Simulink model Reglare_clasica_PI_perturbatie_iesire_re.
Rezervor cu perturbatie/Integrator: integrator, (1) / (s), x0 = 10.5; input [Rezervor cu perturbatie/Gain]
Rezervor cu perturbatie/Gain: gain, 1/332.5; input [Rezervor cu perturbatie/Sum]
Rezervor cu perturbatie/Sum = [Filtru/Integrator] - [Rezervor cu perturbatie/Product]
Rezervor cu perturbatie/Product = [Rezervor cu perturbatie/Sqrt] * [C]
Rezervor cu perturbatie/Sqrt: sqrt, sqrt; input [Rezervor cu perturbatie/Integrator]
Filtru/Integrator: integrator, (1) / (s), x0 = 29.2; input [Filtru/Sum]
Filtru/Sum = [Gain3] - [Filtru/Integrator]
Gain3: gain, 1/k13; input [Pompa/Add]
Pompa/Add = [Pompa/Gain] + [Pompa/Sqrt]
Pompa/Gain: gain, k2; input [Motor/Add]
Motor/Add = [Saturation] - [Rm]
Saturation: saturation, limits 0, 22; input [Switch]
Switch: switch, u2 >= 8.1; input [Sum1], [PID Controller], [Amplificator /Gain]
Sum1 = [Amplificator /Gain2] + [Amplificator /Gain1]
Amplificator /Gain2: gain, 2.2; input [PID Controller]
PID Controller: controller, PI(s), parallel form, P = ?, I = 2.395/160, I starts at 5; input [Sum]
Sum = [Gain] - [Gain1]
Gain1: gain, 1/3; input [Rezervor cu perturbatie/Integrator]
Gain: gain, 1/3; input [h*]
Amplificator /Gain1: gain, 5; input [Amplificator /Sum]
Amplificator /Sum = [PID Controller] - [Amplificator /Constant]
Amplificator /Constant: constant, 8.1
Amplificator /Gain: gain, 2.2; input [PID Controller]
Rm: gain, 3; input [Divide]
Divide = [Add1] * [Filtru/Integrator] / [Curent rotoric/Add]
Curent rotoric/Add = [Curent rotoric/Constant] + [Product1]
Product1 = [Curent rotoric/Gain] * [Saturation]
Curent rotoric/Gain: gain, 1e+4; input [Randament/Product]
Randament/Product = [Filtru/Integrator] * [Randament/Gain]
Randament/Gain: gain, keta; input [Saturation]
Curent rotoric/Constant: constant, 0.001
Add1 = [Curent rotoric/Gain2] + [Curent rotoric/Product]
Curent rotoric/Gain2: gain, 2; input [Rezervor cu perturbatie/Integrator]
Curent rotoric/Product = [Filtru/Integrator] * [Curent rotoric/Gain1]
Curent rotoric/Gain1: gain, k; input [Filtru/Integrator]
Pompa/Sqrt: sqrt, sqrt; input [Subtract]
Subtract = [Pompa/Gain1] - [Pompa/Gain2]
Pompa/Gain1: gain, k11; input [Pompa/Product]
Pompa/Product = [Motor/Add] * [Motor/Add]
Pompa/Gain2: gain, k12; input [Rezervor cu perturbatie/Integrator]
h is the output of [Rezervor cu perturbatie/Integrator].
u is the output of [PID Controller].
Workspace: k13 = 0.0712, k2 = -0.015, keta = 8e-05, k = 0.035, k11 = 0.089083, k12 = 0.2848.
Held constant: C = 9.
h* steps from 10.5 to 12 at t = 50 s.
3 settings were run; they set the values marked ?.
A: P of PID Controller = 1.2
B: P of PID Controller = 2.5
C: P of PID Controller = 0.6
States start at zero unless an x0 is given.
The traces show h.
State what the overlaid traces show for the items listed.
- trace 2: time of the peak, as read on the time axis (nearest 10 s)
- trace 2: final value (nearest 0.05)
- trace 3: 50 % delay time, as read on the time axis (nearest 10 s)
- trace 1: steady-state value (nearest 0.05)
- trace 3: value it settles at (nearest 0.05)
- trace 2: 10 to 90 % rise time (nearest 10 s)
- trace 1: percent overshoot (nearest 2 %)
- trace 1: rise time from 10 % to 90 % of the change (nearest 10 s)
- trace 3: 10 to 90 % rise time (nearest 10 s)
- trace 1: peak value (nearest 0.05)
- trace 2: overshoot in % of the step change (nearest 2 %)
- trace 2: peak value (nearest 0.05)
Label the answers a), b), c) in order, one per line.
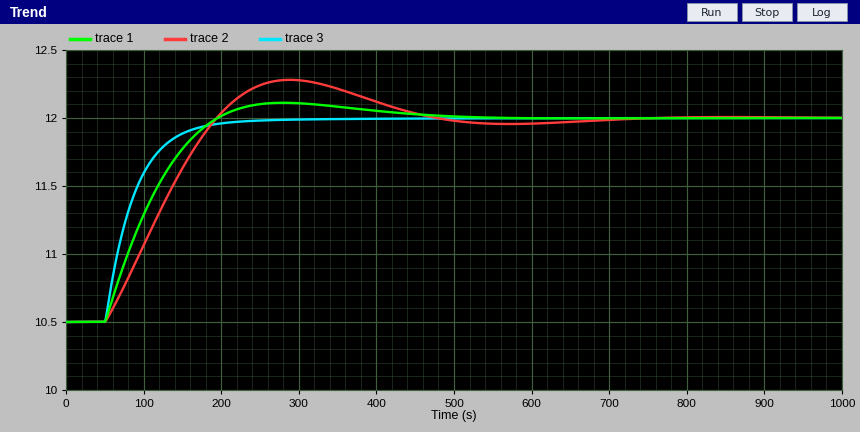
a) 290 s
b) 12.00
c) 80 s
d) 12.00
e) 12.00
f) 110 s
g) 8 %
h) 100 s
i) 80 s
j) 12.10
k) 18 %
l) 12.30
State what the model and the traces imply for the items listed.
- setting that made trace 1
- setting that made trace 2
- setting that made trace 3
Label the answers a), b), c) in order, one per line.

a) A
b) C
c) B
